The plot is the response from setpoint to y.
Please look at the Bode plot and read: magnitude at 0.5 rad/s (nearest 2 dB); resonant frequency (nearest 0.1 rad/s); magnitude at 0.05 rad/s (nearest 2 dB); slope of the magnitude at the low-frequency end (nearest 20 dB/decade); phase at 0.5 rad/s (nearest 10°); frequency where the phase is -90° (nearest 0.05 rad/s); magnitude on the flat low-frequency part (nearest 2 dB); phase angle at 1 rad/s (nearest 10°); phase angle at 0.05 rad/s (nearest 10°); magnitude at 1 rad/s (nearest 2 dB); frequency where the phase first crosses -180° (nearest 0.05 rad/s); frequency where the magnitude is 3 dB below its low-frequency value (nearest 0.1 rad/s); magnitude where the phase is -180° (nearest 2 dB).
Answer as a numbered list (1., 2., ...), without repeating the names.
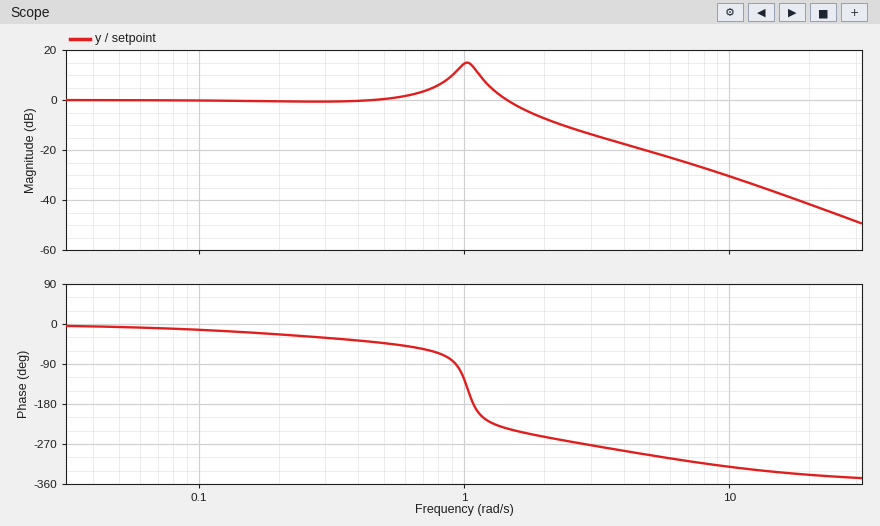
1. 0 dB
2. 1.0 rad/s
3. 0 dB
4. 0 dB/decade
5. -40°
6. 0.95 rad/s
7. 0 dB
8. -120°
9. -10°
10. 14 dB
11. 1.10 rad/s
12. 1.6 rad/s
13. 14 dB
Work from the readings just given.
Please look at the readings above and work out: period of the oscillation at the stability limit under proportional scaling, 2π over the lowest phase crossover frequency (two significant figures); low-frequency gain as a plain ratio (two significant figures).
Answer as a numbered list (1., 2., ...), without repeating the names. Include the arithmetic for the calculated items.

1. 2π / 1.1 = 5.7 s
2. 10^(0 / 20) = 1.0
